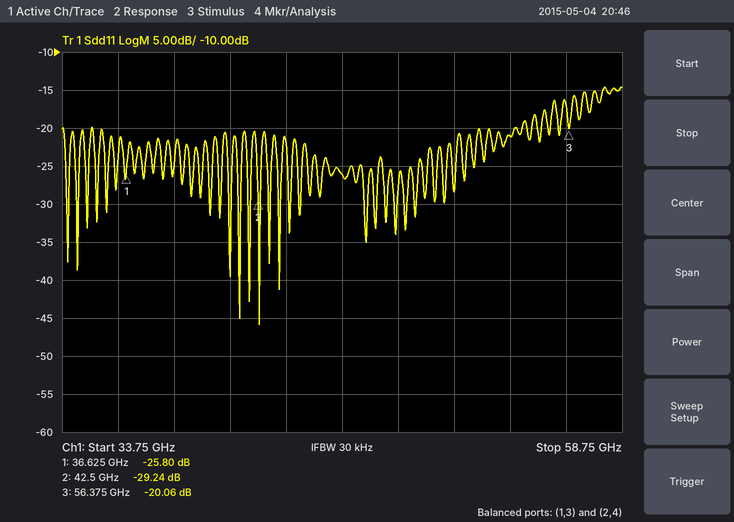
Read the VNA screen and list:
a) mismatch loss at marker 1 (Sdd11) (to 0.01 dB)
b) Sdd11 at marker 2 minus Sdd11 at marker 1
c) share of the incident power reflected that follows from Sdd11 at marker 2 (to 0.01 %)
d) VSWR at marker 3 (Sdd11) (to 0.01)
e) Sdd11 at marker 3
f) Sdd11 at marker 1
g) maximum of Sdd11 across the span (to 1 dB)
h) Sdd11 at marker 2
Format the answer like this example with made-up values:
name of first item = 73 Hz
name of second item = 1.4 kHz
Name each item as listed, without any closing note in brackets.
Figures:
mismatch loss at marker 1 (Sdd11) = 0.01 dB
Sdd11 at marker 2 minus Sdd11 at marker 1 = -3.44 dB
share of the incident power reflected that follows from Sdd11 at marker 2 = 0.12 %
VSWR at marker 3 (Sdd11) = 1.22
Sdd11 at marker 3 = -20.06 dB
Sdd11 at marker 1 = -25.80 dB
maximum of Sdd11 across the span = -15 dB
Sdd11 at marker 2 = -29.24 dB
